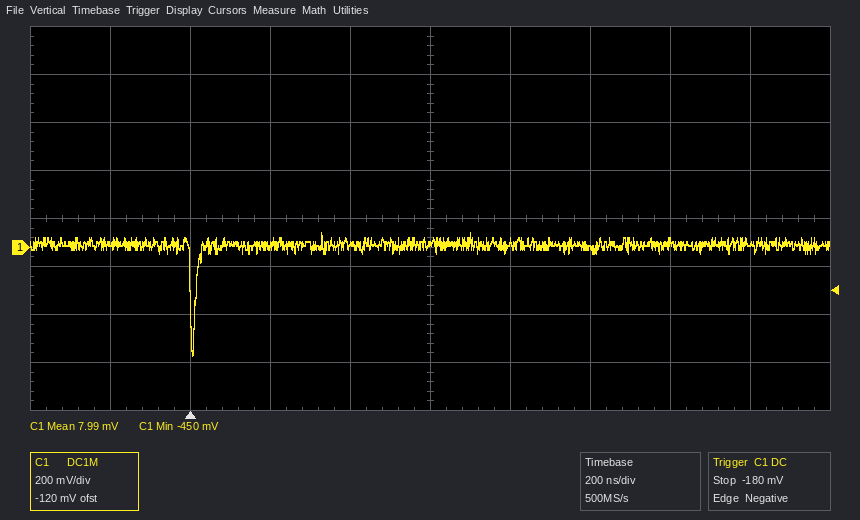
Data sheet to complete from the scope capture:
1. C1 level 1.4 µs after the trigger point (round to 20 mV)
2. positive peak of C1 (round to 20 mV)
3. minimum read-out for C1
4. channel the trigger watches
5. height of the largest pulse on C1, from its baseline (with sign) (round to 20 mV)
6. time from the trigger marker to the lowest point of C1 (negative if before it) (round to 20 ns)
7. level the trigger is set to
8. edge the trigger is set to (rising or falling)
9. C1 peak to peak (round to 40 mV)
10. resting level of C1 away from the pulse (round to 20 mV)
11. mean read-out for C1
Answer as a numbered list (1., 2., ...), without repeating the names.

1. 20 mV
2. 60 mV
3. -450 mV
4. C1
5. -460 mV
6. 0 ns
7. -180 mV
8. falling
9. 520 mV
10. 20 mV
11. 7.99 mV
